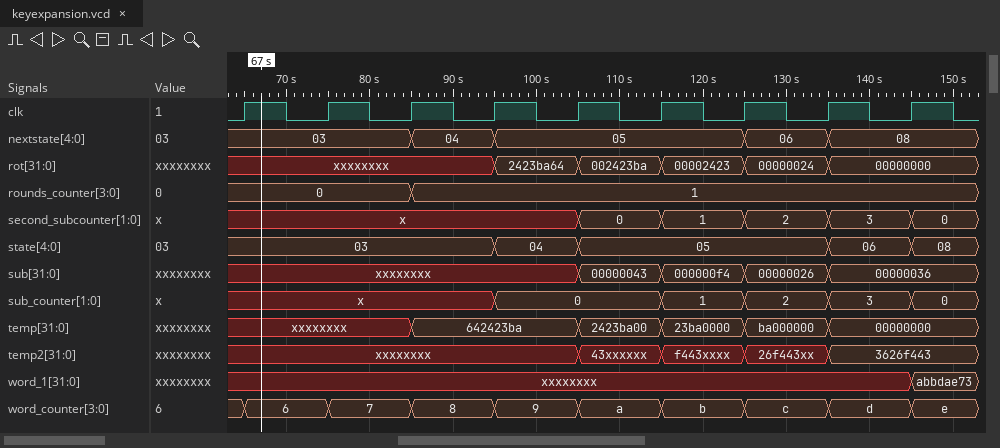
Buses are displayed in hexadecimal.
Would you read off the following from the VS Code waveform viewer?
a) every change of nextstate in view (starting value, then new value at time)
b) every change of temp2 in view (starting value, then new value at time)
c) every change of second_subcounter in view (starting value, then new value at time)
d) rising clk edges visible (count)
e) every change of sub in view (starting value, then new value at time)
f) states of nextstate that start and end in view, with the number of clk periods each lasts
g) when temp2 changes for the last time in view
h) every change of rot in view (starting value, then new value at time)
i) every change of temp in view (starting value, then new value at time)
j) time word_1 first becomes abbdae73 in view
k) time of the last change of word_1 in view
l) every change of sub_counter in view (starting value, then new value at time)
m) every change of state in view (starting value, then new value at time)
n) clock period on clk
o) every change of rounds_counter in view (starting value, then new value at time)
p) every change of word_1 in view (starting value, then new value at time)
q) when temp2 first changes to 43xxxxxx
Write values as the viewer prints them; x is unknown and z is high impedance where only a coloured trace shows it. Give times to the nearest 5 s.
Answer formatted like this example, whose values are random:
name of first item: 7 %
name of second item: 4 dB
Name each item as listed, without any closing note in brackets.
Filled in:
every change of nextstate in view: 03, 04 at 85 s, 05 at 95 s, 06 at 125 s, 08 at 135 s
every change of temp2 in view: xxxxxxxx, 43xxxxxx at 105 s, f443xxxx at 115 s, 26f443xx at 125 s, 3626f443 at 135 s
every change of second_subcounter in view: x, 0 at 105 s, 1 at 115 s, 2 at 125 s, 3 at 135 s, 0 at 145 s
rising clk edges visible: 9
every change of sub in view: xxxxxxxx, 00000043 at 105 s, 000000f4 at 115 s, 00000026 at 125 s, 00000036 at 135 s
states of nextstate that start and end in view, with the number of clk periods each lasts: 04: 1, 05: 3, 06: 1
when temp2 changes for the last time in view: 135 s
every change of rot in view: xxxxxxxx, 2423ba64 at 95 s, 002423ba at 105 s, 00002423 at 115 s, 00000024 at 125 s, 00000000 at 135 s
every change of temp in view: xxxxxxxx, 642423ba at 85 s, 2423ba00 at 105 s, 23ba0000 at 115 s, ba000000 at 125 s, 00000000 at 135 s
time word_1 first becomes abbdae73 in view: 145 s
time of the last change of word_1 in view: 145 s
every change of sub_counter in view: x, 0 at 95 s, 1 at 115 s, 2 at 125 s, 3 at 135 s, 0 at 145 s
every change of state in view: 03, 04 at 95 s, 05 at 105 s, 06 at 135 s, 08 at 145 s
clock period on clk: 10 s
every change of rounds_counter in view: 0, 1 at 85 s
every change of word_1 in view: xxxxxxxx, abbdae73 at 145 s
when temp2 first changes to 43xxxxxx: 105 s
